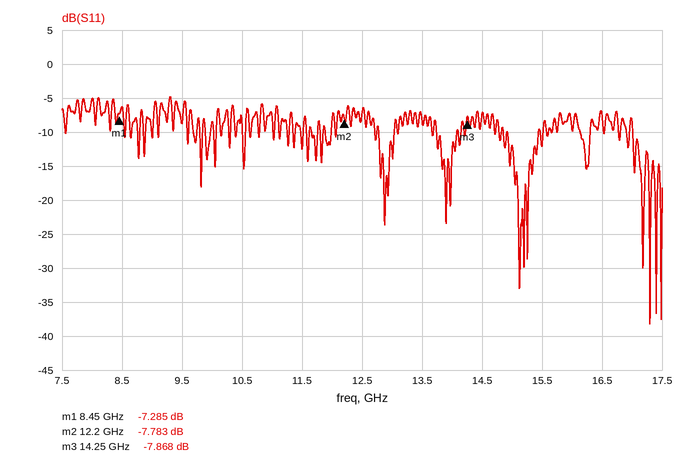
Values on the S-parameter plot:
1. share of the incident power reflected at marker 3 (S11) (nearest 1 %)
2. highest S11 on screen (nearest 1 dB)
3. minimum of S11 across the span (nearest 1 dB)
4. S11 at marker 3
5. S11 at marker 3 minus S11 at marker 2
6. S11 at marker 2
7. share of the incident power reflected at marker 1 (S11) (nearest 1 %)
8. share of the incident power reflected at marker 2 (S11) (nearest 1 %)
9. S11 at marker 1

16 %
-5 dB
-38 dB
-7.868 dB
-0.085 dB
-7.783 dB
19 %
17 %
-7.285 dB
